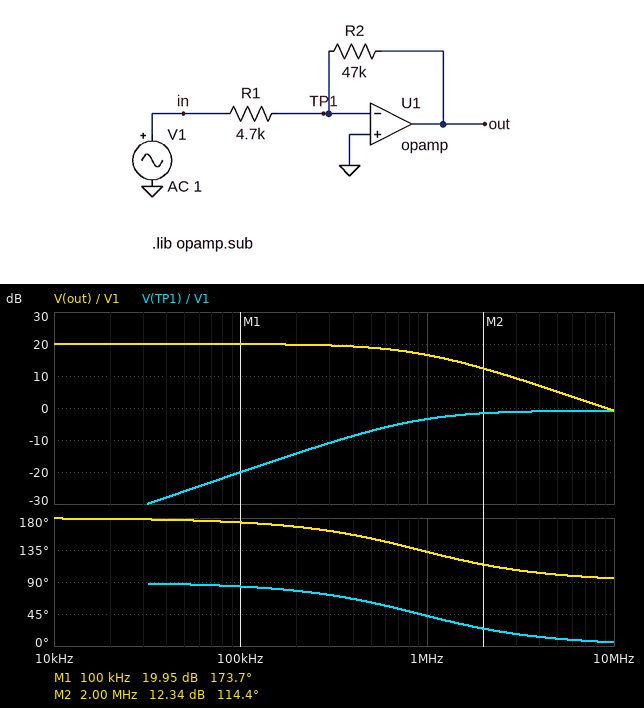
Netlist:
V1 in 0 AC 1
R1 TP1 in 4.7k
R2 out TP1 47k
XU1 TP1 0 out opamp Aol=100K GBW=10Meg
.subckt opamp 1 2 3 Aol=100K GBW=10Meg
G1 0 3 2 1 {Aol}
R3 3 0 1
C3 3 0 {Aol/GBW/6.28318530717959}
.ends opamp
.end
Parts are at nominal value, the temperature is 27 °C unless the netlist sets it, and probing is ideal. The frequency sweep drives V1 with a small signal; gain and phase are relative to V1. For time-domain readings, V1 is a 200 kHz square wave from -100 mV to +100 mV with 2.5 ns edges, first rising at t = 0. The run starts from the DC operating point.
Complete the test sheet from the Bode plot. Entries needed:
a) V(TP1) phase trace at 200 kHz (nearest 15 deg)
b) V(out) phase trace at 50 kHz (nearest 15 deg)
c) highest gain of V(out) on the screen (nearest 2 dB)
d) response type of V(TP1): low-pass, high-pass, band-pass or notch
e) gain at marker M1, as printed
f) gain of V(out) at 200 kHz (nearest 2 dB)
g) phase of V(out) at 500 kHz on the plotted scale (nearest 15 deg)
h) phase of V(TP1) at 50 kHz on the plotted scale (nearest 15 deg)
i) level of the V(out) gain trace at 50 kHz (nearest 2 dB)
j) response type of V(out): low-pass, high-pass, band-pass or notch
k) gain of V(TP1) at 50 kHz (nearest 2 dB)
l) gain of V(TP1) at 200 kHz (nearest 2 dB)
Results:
75 deg
180 deg
20 dB
high-pass
19.95 dB
20 dB
150 deg
90 deg
20 dB
low-pass
-26 dB
-14 dB
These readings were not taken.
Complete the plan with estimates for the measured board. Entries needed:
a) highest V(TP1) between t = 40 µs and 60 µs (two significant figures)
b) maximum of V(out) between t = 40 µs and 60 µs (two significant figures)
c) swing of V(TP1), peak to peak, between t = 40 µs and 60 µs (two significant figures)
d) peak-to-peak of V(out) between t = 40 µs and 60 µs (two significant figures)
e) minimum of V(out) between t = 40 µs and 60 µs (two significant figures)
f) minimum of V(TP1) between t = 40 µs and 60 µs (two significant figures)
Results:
180 mV
1.0 V
360 mV
2.0 V
-1.0 V
-180 mV
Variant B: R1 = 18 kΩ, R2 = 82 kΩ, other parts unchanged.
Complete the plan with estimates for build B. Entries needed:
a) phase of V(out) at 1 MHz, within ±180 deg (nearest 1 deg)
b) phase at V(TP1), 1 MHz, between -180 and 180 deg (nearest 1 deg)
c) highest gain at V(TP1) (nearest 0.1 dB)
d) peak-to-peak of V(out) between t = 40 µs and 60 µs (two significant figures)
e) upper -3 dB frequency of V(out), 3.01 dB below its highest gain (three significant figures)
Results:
151 deg
61 deg
-1.7 dB
910 mV
1.80 MHz
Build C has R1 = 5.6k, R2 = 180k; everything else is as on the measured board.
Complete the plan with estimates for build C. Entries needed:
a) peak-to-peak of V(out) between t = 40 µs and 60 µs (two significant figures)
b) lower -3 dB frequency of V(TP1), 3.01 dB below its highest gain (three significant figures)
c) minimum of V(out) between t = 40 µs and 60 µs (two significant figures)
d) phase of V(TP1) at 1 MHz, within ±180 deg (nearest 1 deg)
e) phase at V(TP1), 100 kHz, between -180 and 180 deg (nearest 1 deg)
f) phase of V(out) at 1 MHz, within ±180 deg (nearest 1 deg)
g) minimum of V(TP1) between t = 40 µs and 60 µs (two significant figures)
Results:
6.3 V
302 kHz
-3.2 V
17 deg
72 deg
107 deg
-190 mV
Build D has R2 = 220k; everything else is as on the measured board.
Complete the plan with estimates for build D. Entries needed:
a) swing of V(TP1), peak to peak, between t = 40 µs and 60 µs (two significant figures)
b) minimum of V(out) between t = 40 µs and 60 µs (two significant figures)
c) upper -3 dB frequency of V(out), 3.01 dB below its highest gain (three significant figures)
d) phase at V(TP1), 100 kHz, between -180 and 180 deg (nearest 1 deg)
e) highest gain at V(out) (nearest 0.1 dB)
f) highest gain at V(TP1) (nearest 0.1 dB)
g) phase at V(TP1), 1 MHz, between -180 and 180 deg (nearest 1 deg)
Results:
380 mV
-4.3 V
209 kHz
64 deg
33.4 dB
-0.2 dB
12 deg
